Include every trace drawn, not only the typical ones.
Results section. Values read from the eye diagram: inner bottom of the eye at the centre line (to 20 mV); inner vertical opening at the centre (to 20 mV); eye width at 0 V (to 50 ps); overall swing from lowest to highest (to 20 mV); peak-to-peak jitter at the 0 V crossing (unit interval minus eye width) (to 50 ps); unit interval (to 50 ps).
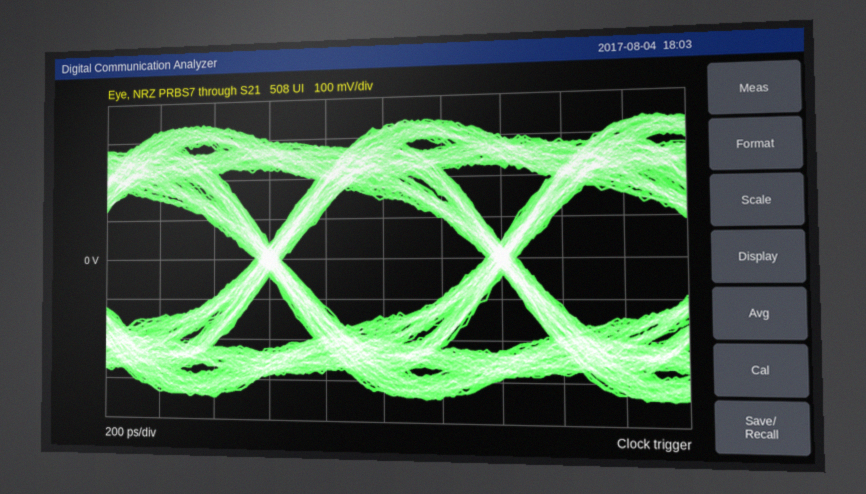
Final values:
-140 mV
300 mV
700 ps
680 mV
100 ps
800 ps
